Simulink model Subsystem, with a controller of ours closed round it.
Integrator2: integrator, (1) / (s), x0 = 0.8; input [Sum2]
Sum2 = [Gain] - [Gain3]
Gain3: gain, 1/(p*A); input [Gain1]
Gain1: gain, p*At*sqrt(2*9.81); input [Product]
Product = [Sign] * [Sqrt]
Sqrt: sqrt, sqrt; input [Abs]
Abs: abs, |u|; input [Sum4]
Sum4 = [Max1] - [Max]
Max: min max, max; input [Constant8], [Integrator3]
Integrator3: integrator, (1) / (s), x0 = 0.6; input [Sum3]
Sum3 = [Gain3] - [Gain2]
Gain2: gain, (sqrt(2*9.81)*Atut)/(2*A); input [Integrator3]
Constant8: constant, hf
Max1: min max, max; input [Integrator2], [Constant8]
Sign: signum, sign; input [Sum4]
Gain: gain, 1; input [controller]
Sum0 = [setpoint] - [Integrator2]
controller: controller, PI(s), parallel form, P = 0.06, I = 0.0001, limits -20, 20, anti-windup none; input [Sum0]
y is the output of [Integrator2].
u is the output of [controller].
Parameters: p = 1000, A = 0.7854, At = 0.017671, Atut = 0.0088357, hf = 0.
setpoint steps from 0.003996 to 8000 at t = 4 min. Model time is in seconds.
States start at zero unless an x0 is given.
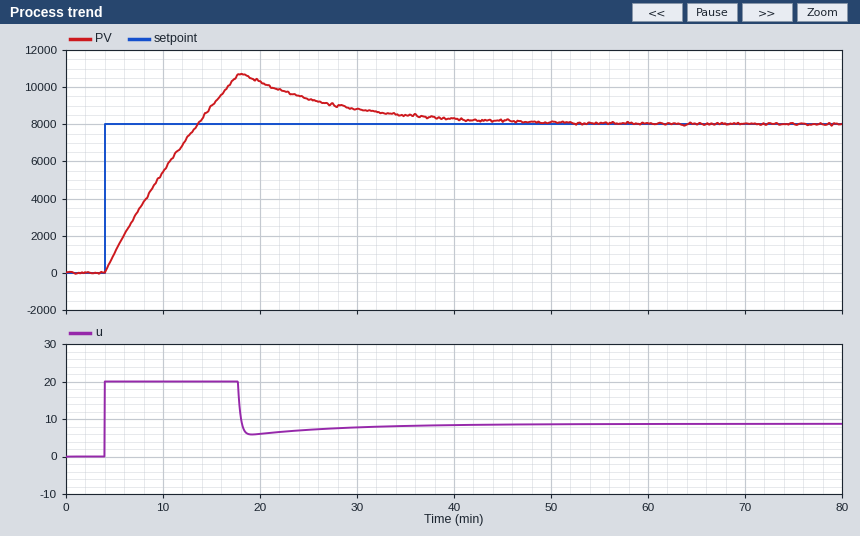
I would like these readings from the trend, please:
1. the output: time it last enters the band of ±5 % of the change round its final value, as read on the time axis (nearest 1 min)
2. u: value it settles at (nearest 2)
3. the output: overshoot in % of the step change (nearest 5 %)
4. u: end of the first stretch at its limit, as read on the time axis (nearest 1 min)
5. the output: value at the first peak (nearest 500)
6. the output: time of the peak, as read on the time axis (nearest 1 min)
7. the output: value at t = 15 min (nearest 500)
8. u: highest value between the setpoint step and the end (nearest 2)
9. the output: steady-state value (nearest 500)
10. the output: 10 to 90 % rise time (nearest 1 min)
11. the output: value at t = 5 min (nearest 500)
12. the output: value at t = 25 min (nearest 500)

37 min
8
35 %
18 min
10500
18 min
9000
20
8000
8 min
1000
9500
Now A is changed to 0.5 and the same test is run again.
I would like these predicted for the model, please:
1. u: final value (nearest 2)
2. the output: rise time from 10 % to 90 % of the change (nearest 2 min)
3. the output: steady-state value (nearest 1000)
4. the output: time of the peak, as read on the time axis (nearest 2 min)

14
10 min
8000
26 min
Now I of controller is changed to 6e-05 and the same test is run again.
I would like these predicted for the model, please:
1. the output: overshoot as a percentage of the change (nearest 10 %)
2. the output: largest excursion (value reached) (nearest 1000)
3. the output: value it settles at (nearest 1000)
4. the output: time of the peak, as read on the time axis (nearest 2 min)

20 %
10000
8000
16 min
